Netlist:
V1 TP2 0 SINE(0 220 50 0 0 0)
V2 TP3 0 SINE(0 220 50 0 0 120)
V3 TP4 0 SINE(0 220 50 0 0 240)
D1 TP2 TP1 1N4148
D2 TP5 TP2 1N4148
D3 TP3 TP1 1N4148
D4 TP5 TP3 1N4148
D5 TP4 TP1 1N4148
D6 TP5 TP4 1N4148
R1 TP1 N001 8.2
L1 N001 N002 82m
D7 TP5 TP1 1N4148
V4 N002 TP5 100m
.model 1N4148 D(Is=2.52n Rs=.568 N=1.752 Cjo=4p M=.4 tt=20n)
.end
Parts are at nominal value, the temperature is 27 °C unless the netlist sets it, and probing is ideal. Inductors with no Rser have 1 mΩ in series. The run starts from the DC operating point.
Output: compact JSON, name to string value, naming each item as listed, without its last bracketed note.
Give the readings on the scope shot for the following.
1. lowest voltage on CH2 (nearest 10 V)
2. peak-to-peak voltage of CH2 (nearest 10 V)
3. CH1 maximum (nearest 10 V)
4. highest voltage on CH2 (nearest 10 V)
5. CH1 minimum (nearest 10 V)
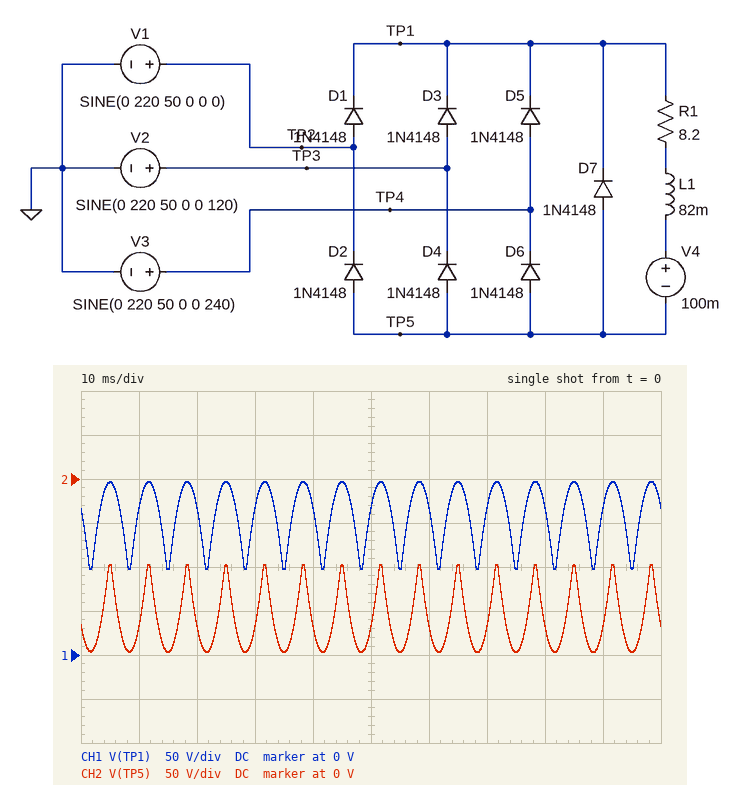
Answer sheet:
{"lowest voltage on CH2": "-200 V", "peak-to-peak voltage of CH2": "100 V", "CH1 maximum": "200 V", "highest voltage on CH2": "-100 V", "CH1 minimum": "100 V"}
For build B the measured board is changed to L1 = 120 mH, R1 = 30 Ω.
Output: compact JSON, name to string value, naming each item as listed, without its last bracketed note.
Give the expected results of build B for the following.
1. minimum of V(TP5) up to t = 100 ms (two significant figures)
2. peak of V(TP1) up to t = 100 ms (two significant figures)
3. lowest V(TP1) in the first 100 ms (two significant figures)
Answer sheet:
{"minimum of V(TP5) up to t = 100 ms": "-210 V", "peak of V(TP1) up to t = 100 ms": "210 V", "lowest V(TP1) in the first 100 ms": "110 V"}
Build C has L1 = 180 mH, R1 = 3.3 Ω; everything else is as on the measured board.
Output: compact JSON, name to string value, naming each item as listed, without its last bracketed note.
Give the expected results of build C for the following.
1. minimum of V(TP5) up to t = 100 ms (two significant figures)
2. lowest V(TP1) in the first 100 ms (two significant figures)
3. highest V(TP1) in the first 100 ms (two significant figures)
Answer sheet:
{"minimum of V(TP5) up to t = 100 ms": "-170 V", "lowest V(TP1) in the first 100 ms": "84 V", "highest V(TP1) in the first 100 ms": "170 V"}
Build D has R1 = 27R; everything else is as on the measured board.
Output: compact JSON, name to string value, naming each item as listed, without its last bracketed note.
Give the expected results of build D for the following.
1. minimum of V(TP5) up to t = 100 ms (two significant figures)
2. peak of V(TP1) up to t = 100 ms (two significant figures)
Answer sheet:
{"minimum of V(TP5) up to t = 100 ms": "-210 V", "peak of V(TP1) up to t = 100 ms": "210 V"}
